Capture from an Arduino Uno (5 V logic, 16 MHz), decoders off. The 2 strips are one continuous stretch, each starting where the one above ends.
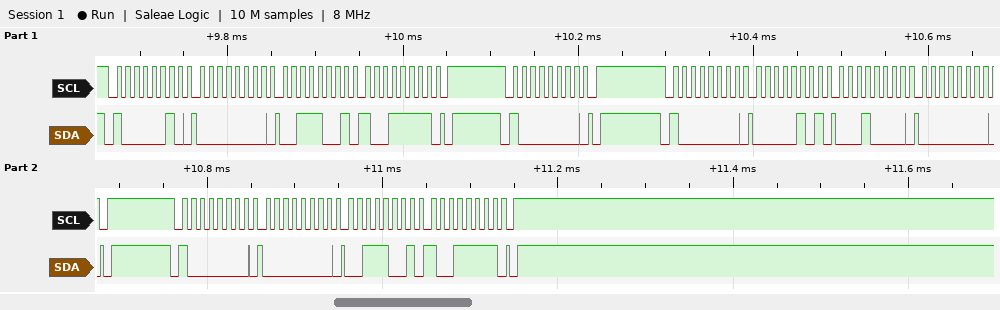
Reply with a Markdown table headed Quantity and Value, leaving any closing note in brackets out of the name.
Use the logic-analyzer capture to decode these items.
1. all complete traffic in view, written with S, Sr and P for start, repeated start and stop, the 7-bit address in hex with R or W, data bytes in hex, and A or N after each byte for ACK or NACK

| Quantity | Value |
|---|---|
| all complete traffic in view, written with S, Sr and P for start, repeated start and stop, the 7-bit address in hex with R or W, data bytes in hex, and A or N after each byte for ACK or NACK | S 41W A 00 A 39 A 9F A P S 40W A P S 40W A 05 A 10 A 00 A P S 40W A 00 A 39 A 9F A P |
